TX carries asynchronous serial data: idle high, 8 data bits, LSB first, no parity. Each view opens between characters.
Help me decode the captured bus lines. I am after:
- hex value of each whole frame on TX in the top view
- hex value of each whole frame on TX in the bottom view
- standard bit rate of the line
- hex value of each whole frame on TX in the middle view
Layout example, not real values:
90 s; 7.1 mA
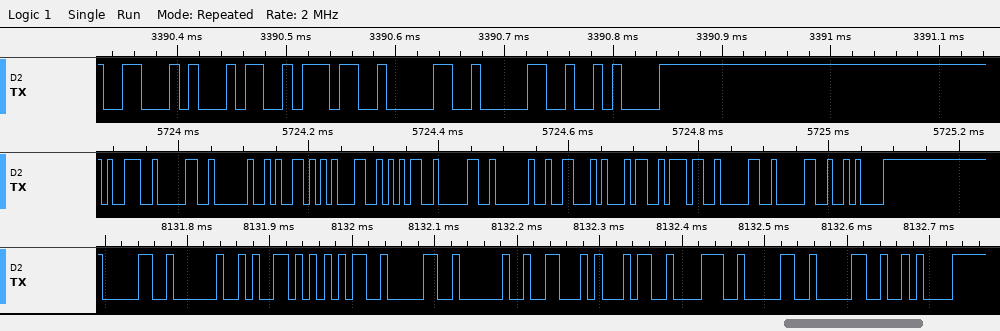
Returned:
46, 34, 37, 30, 30, 0A; 30, 20, 59, 35, 30, 20, 46, 34, 38, 30, 30, 0A; 115200 baud; 39, 30, 20, 59, 31, 35, 30, 20, 46, 34, 37, 30, 30, 0A
